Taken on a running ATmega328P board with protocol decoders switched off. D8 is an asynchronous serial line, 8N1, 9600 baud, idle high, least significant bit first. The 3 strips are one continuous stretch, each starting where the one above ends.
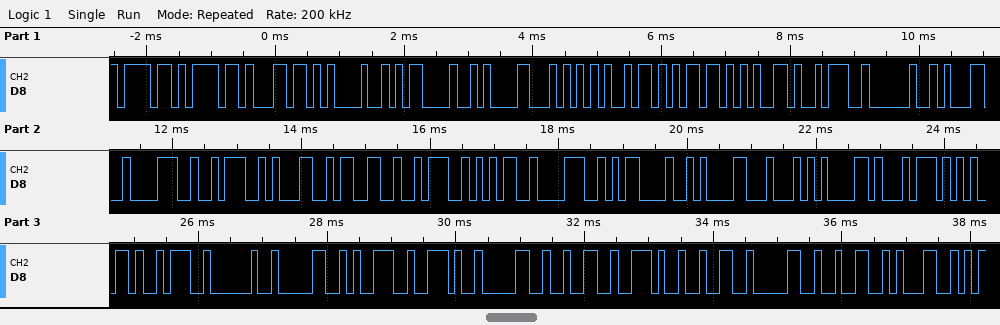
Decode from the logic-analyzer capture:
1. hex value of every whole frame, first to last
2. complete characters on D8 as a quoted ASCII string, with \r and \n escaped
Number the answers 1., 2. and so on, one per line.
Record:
1. 6F 6F 6C 21 0D 0A 54 69 6D 65 3A 20 31 38 3A 31 33 3A 35 38 0D 0A 44 61 74 65 3A 20 30 39 2E 30 32 2E 32 30 32 31
2. "ool!\r\nTime: 18:13:58\r\nDate: 09.02.2021"
